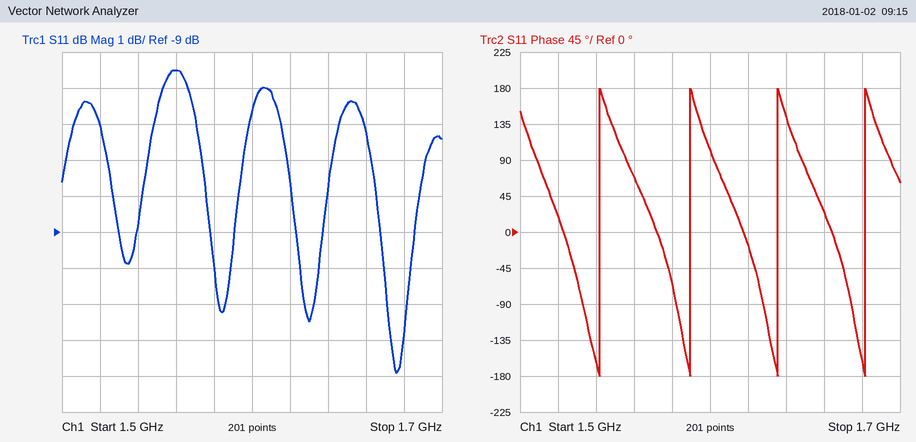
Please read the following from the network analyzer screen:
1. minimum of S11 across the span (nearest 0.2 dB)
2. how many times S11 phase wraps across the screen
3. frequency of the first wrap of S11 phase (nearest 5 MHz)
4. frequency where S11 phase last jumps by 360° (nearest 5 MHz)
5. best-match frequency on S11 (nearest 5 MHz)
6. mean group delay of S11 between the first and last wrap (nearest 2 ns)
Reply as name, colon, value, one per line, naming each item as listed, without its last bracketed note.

minimum of S11 across the span: -13.0 dB
how many times S11 phase wraps across the screen: 4
frequency of the first wrap of S11 phase: 1.540 GHz
frequency where S11 phase last jumps by 360°: 1.680 GHz
best-match frequency on S11: 1.675 GHz
mean group delay of S11 between the first and last wrap: 22 ns
